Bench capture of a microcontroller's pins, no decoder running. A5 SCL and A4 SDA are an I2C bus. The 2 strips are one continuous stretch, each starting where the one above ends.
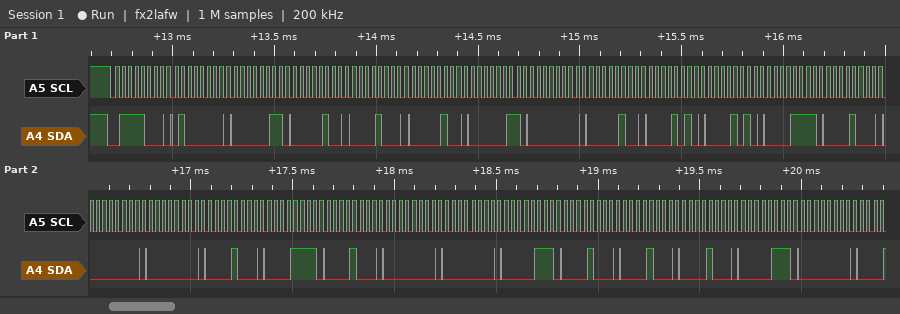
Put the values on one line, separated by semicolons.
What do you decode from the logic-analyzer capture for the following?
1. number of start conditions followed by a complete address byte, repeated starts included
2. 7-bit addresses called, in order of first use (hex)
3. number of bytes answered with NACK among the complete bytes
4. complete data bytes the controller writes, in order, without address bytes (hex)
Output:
1; 0x3C; 0; 40 03 04 08 04 03 00 04 0A 0A 0F 08 00 00 08 0F 08 00 00 07 08 08 08 07 00
